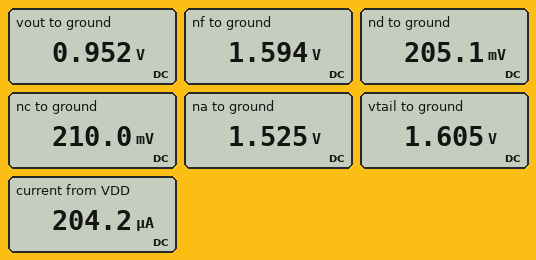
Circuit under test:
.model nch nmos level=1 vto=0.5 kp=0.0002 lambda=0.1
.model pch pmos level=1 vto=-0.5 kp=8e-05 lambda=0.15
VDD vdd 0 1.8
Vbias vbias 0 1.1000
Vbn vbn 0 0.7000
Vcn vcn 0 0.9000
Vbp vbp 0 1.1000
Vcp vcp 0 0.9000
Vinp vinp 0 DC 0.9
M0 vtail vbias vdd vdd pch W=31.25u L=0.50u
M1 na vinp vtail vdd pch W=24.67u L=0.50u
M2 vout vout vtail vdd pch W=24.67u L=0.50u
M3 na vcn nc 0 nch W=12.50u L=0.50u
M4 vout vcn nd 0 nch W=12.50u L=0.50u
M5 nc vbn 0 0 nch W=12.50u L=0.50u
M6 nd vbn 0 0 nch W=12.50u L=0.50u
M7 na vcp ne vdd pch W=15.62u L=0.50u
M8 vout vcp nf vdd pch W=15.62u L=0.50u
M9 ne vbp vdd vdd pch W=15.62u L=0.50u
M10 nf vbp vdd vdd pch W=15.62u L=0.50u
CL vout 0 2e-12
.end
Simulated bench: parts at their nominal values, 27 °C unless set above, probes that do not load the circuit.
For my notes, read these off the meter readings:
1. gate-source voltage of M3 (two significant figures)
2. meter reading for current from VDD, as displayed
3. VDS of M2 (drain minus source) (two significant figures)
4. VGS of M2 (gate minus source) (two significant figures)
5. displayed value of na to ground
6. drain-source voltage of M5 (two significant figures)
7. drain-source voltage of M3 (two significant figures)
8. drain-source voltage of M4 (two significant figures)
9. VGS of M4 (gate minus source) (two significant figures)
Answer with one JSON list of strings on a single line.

["690 mV", "204.2 µA", "-650 mV", "-650 mV", "1.525 V", "210 mV", "1.3 V", "750 mV", "690 mV"]
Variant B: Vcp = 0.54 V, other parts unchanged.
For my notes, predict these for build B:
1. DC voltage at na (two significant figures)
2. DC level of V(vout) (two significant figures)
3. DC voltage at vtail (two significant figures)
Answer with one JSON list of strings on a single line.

["1.6 V", "990 mV", "1.6 V"]
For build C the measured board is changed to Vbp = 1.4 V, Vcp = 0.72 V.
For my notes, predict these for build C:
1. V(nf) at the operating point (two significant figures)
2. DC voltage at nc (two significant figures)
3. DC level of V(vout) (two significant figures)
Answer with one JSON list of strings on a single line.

["1.2 V", "3.4 mV", "720 mV"]
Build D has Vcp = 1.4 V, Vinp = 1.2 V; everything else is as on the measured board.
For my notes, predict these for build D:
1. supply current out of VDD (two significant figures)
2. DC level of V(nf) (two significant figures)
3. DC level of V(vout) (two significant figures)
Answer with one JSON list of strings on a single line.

["100 µA", "1.8 V", "900 mV"]
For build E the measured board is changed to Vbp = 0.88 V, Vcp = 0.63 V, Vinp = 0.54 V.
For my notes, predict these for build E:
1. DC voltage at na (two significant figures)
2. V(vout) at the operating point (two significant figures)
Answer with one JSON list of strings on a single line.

["1.7 V", "1.6 V"]
